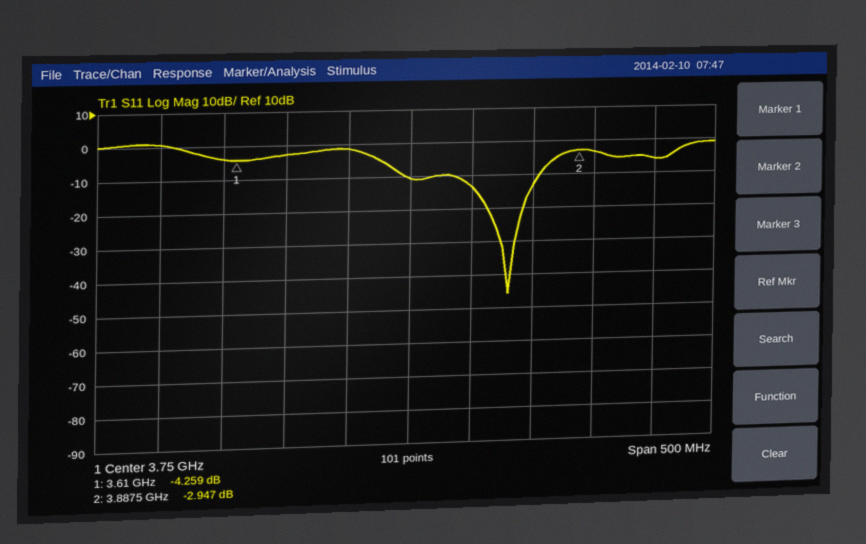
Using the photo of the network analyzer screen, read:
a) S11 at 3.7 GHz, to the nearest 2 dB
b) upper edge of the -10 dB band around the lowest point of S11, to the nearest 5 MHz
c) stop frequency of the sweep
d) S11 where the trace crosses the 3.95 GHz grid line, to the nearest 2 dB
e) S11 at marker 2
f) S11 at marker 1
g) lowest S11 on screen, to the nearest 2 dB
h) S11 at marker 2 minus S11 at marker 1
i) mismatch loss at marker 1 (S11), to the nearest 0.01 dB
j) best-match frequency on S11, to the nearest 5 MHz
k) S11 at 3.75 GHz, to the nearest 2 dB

-2 dB
3.855 GHz
4 GHz
-6 dB
-2.947 dB
-4.259 dB
-46 dB
1.312 dB
2.04 dB
3.830 GHz
-10 dB
